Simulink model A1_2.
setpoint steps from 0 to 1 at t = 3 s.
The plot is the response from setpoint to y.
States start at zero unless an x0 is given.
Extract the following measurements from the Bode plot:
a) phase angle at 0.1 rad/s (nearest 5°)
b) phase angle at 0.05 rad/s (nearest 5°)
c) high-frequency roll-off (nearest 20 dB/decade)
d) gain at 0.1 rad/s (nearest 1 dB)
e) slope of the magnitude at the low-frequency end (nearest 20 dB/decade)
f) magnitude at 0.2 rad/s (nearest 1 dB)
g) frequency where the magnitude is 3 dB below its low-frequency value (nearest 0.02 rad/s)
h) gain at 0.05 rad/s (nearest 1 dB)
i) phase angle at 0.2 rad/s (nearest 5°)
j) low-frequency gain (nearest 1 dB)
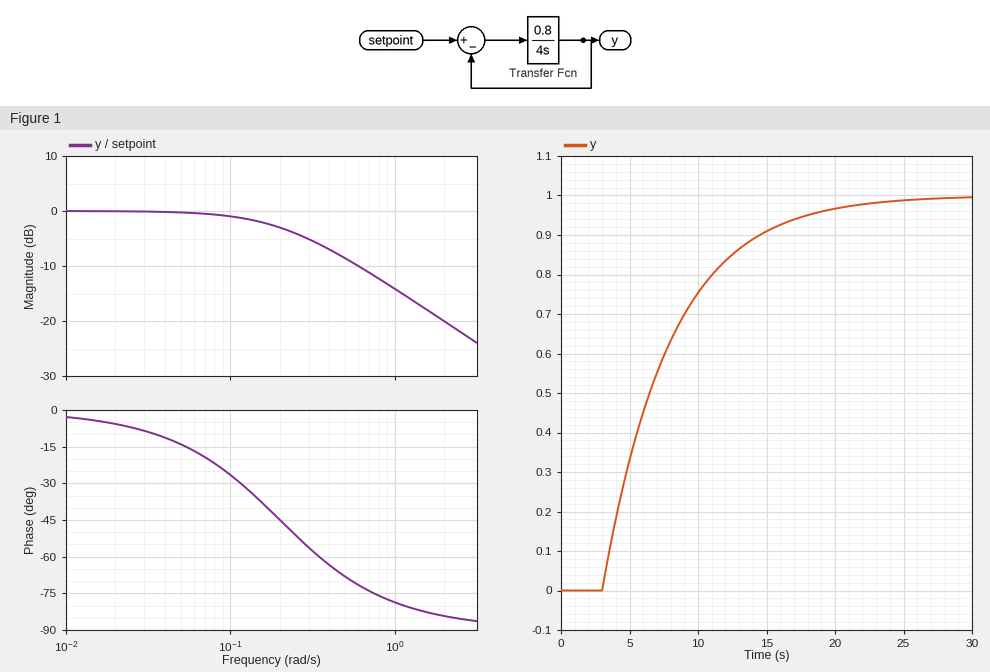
-25°
-15°
-20 dB/decade
-1 dB
0 dB/decade
-3 dB
0.20 rad/s
0 dB
-45°
0 dB
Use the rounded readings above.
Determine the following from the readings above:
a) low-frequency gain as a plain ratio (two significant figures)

1.0
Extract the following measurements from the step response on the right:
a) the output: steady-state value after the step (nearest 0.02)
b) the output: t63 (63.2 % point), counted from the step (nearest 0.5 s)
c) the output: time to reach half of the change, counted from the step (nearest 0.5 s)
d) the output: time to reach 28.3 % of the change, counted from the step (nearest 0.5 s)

1.00
5.0 s
3.5 s
1.5 s
